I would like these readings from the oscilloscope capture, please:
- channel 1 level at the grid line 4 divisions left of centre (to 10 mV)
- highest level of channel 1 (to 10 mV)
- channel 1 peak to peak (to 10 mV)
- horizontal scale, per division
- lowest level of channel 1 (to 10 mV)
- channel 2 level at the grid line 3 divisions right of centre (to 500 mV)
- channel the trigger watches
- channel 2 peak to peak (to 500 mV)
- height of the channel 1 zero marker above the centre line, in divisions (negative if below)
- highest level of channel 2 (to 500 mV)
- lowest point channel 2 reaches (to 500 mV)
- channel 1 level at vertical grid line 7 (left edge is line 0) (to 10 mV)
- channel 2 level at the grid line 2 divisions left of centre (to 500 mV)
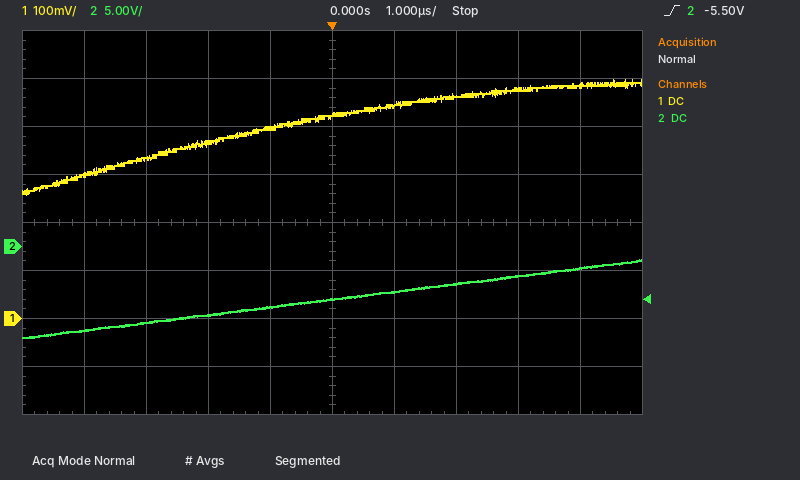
300 mV
500 mV
240 mV
1 µs
260 mV
-3.0 V
channel 2
8.0 V
-2.0 div
-1.5 V
-9.5 V
460 mV
-7.0 V
